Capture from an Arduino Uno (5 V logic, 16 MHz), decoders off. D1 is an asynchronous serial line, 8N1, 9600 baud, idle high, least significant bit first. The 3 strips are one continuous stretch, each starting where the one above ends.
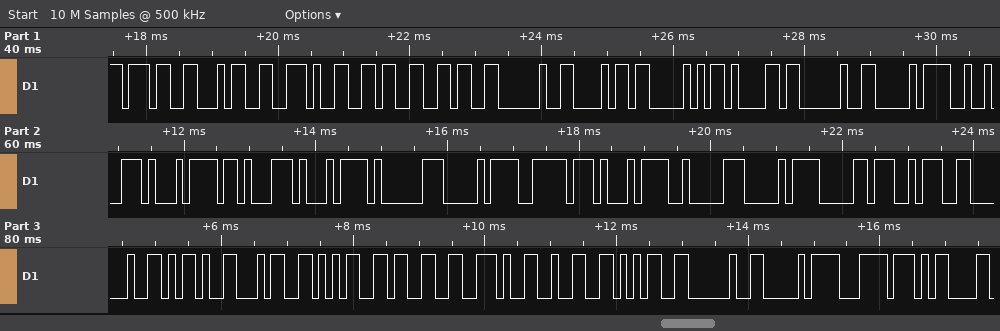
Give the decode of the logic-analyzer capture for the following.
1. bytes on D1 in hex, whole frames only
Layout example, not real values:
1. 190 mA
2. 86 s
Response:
1. 37 34 2E 36 36 20 68 50 61 20 D0 92 D1 8B D1 81 D0 BE D1 82 D0 B0 3A 20 2D 34 35 33 2E 32 35 20 D0 BC 0D
